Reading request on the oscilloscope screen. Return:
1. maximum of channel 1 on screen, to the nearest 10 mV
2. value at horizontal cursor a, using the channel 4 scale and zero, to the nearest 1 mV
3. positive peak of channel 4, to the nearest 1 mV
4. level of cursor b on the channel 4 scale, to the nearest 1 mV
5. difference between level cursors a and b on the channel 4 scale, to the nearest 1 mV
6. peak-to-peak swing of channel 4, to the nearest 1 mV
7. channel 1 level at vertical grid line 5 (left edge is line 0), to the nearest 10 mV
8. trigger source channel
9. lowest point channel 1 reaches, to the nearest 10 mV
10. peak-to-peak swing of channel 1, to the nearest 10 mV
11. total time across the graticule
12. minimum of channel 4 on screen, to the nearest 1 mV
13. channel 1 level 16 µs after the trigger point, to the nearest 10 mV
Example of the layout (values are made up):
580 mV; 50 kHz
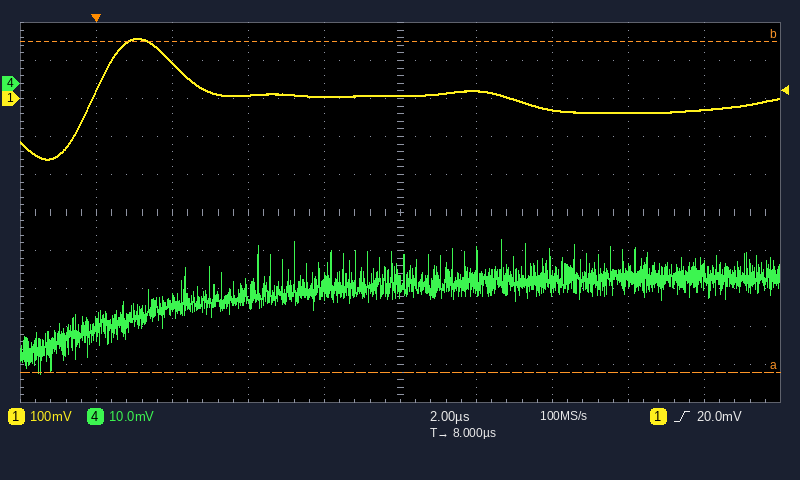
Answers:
160 mV; -76 mV; -41 mV; 11 mV; 87 mV; 35 mV; 10 mV; channel 1; -160 mV; 320 mV; 20 µs; -76 mV; -30 mV
